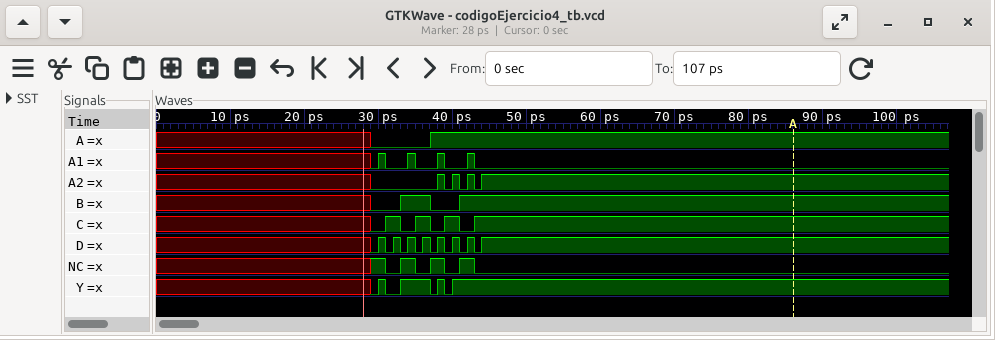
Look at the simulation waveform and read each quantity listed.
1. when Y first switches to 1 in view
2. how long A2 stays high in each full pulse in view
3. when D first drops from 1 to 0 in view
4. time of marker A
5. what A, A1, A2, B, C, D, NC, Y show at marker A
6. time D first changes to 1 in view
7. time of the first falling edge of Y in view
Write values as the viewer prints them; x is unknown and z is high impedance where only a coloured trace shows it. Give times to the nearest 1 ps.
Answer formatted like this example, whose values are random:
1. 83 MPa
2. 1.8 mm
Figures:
1. 30 ps
2. 1 ps, 1 ps, 1 ps
3. 31 ps
4. 86 ps
5. A=1, A1=0, A2=1, B=1, C=1, D=1, NC=0, Y=1
6. 30 ps
7. 31 ps
